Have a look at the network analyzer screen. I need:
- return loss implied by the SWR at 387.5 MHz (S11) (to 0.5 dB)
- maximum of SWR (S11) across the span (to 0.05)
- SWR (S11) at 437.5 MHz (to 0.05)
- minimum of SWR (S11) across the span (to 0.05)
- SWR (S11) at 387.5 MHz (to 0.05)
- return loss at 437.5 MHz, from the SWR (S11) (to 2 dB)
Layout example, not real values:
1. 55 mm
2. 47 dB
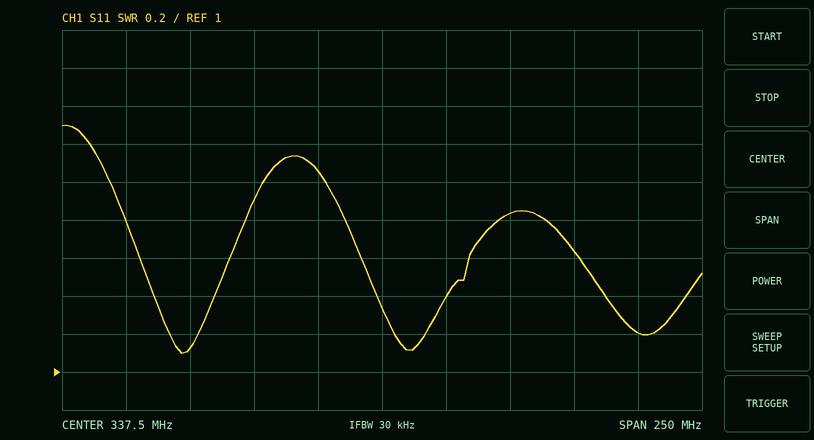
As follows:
1. 10.5 dB
2. 2.30
3. 1.20
4. 1.10
5. 1.85
6. 20 dB
